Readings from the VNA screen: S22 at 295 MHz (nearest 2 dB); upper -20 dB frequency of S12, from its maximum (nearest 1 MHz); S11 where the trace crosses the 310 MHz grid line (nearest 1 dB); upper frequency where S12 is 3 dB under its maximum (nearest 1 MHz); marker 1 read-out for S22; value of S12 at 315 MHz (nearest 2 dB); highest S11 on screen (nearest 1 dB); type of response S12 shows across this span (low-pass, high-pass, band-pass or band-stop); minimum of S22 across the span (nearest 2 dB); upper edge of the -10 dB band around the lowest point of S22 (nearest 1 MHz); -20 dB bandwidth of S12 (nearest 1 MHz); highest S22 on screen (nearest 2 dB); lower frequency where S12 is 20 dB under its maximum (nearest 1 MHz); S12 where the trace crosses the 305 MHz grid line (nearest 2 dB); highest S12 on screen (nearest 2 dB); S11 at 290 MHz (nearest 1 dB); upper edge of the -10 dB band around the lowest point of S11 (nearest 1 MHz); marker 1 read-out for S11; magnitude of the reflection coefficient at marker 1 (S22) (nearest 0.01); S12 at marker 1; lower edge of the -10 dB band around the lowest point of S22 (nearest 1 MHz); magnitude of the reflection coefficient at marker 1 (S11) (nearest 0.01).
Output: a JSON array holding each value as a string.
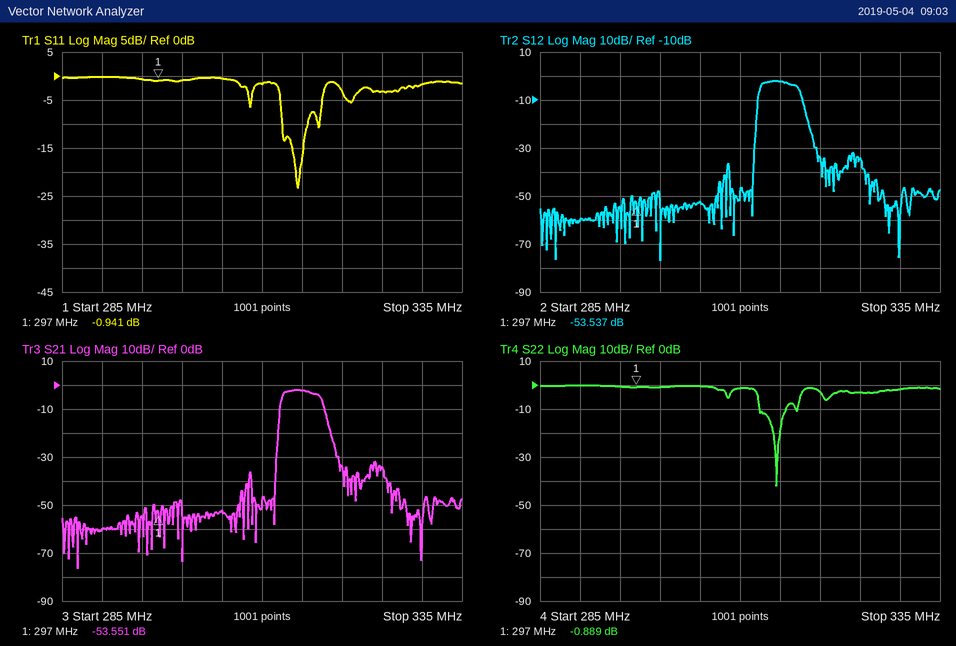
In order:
["0 dB", "319 MHz", "-2 dB", "317 MHz", "-0.889 dB", "-2 dB", "0 dB", "band-pass", "-42 dB", "316 MHz", "7 MHz", "0 dB", "312 MHz", "-52 dB", "-2 dB", "0 dB", "316 MHz", "-0.941 dB", "0.90", "-53.537 dB", "312 MHz", "0.90"]
